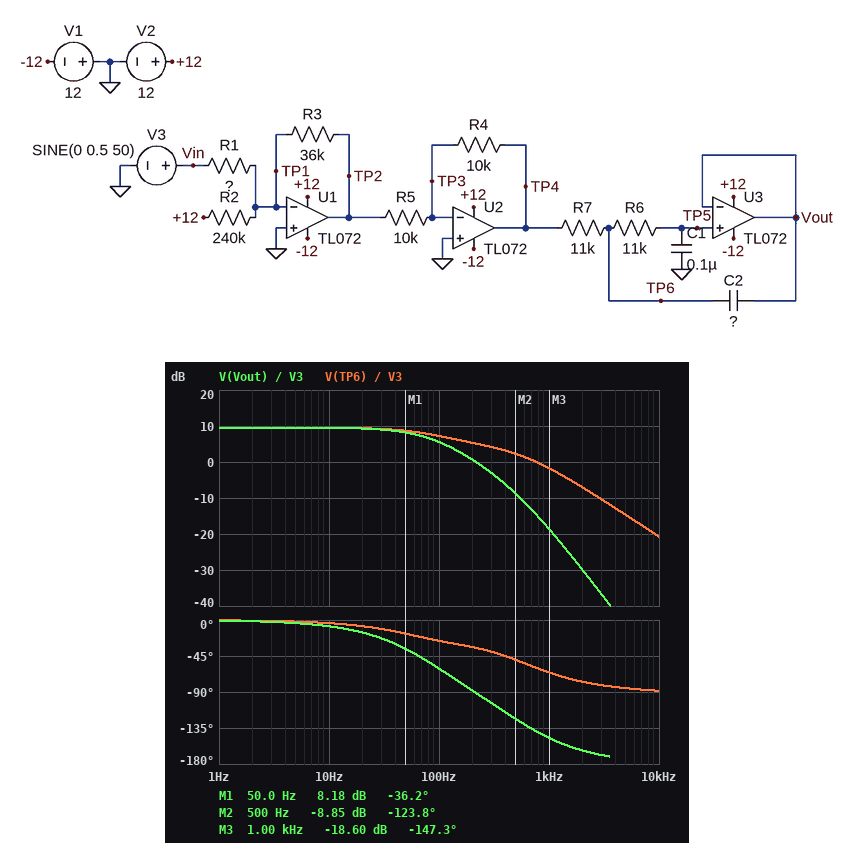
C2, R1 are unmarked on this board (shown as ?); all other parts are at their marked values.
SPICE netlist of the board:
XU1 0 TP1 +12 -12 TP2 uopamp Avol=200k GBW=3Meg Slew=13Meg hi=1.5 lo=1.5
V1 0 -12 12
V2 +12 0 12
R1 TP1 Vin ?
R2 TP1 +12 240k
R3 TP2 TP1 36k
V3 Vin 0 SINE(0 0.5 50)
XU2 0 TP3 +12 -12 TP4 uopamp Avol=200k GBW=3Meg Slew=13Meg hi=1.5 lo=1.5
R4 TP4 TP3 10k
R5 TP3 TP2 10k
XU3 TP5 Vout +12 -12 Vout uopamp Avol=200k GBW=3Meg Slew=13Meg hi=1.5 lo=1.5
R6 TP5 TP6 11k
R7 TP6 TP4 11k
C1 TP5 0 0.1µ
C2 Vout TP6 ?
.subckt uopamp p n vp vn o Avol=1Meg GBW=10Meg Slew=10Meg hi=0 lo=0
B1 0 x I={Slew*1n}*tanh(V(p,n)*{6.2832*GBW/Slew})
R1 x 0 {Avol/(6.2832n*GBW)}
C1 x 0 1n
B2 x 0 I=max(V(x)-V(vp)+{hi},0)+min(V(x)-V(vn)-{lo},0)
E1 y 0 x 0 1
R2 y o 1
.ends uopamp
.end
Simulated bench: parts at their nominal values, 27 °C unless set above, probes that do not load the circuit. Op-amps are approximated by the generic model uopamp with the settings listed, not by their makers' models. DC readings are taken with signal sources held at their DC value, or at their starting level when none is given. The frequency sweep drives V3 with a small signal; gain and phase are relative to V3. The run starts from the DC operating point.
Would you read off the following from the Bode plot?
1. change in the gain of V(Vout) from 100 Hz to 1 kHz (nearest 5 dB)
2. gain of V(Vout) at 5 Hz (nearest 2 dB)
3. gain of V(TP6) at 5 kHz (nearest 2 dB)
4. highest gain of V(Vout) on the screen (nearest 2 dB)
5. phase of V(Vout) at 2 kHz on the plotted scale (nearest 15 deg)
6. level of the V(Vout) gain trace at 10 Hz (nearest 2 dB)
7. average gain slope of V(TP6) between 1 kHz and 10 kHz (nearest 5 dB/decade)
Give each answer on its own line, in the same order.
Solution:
-25 dB
10 dB
-14 dB
10 dB
-165 deg
10 dB
-20 dB/decade
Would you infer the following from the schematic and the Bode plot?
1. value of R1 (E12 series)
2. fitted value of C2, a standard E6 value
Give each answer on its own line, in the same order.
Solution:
12 kΩ
47 nF
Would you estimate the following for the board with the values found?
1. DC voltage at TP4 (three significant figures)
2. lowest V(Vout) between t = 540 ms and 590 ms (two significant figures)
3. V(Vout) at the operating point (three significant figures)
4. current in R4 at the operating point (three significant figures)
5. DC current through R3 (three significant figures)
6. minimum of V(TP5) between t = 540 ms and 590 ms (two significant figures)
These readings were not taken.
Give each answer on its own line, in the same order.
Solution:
1.80 V
520 mV
1.80 V
180 µA
50.0 µA
520 mV
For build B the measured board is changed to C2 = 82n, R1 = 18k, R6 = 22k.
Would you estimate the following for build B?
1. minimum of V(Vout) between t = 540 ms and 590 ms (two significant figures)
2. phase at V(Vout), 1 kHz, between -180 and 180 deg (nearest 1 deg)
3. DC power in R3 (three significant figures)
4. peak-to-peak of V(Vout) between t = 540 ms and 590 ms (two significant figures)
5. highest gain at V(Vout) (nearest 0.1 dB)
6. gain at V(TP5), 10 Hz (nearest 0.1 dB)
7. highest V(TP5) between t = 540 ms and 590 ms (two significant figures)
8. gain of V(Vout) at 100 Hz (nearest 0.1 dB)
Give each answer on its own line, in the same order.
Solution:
1.0 V
-165 deg
90.0 µW
1.5 V
6.0 dB
5.9 dB
2.6 V
-0.4 dB
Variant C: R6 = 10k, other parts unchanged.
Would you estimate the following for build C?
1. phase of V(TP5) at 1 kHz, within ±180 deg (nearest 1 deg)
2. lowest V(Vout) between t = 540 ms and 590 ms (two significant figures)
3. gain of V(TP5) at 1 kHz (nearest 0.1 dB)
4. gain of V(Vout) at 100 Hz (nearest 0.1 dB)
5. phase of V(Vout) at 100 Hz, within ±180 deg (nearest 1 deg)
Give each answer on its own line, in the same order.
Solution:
-146 deg
500 mV
-17.9 dB
5.8 dB
-59 deg
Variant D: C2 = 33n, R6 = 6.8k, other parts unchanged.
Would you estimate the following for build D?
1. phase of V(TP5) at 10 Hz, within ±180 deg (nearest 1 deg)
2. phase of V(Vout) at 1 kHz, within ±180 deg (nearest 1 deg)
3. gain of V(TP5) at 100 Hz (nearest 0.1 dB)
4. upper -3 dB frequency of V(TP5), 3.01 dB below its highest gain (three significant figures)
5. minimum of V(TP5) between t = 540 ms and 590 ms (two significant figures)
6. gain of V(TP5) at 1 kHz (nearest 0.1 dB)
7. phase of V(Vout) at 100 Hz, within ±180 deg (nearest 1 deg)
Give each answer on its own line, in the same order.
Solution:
-6 deg
-128 deg
6.4 dB
96.9 Hz
470 mV
-13.5 dB
-51 deg
